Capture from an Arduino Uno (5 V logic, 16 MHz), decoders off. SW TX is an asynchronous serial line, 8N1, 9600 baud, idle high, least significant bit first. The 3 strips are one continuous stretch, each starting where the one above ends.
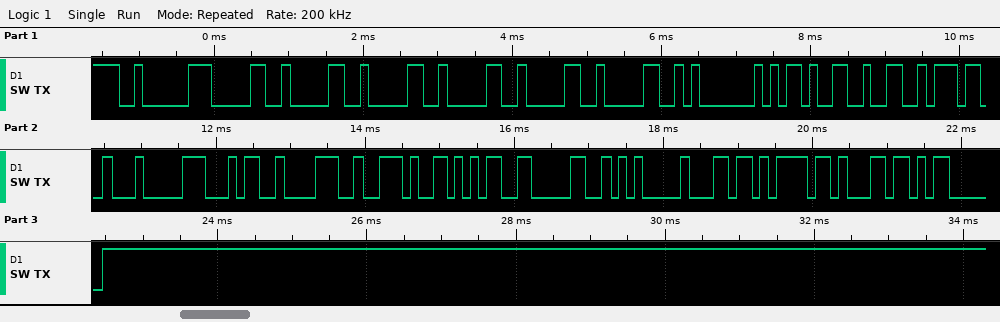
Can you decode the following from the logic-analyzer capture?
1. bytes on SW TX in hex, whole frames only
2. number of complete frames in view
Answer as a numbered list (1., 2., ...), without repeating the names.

1. 02 30 30 30 30 30 30 01 2D 32 37 04 34 38 2E 35 30 05 6C 6F 6C 03
2. 22
